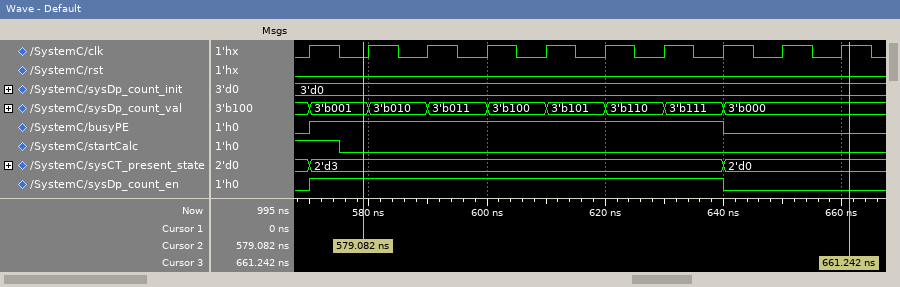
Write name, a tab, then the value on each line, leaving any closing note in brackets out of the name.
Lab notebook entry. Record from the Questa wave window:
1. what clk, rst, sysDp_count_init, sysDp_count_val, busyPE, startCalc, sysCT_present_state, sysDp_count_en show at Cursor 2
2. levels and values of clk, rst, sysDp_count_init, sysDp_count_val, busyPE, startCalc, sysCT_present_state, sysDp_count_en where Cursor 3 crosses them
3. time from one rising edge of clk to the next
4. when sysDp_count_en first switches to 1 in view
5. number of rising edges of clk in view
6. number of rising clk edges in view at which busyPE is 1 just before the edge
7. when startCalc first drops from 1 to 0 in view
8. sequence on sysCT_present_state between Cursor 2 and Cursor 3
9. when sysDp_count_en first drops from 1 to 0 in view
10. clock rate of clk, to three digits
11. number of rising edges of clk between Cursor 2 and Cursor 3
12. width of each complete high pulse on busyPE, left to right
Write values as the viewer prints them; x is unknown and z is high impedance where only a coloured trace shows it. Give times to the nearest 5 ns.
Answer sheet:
what clk, rst, sysDp_count_init, sysDp_count_val, busyPE, startCalc, sysCT_present_state, sysDp_count_en show at Cursor 2	clk=0, rst=0, sysDp_count_init=3'd0, sysDp_count_val=3'b001, busyPE=1, startCalc=0, sysCT_present_state=2'd3, sysDp_count_en=1
levels and values of clk, rst, sysDp_count_init, sysDp_count_val, busyPE, startCalc, sysCT_present_state, sysDp_count_en where Cursor 3 crosses them	clk=1, rst=0, sysDp_count_init=3'd0, sysDp_count_val=3'b000, busyPE=0, startCalc=0, sysCT_present_state=2'd0, sysDp_count_en=0
time from one rising edge of clk to the next	10 ns
when sysDp_count_en first switches to 1 in view	570 ns
number of rising edges of clk in view	10
number of rising clk edges in view at which busyPE is 1 just before the edge	7
when startCalc first drops from 1 to 0 in view	575 ns
sequence on sysCT_present_state between Cursor 2 and Cursor 3	2'd3, 2'd0
when sysDp_count_en first drops from 1 to 0 in view	640 ns
clock rate of clk, to three digits	100 MHz
number of rising edges of clk between Cursor 2 and Cursor 3	9
width of each complete high pulse on busyPE, left to right	70 ns
